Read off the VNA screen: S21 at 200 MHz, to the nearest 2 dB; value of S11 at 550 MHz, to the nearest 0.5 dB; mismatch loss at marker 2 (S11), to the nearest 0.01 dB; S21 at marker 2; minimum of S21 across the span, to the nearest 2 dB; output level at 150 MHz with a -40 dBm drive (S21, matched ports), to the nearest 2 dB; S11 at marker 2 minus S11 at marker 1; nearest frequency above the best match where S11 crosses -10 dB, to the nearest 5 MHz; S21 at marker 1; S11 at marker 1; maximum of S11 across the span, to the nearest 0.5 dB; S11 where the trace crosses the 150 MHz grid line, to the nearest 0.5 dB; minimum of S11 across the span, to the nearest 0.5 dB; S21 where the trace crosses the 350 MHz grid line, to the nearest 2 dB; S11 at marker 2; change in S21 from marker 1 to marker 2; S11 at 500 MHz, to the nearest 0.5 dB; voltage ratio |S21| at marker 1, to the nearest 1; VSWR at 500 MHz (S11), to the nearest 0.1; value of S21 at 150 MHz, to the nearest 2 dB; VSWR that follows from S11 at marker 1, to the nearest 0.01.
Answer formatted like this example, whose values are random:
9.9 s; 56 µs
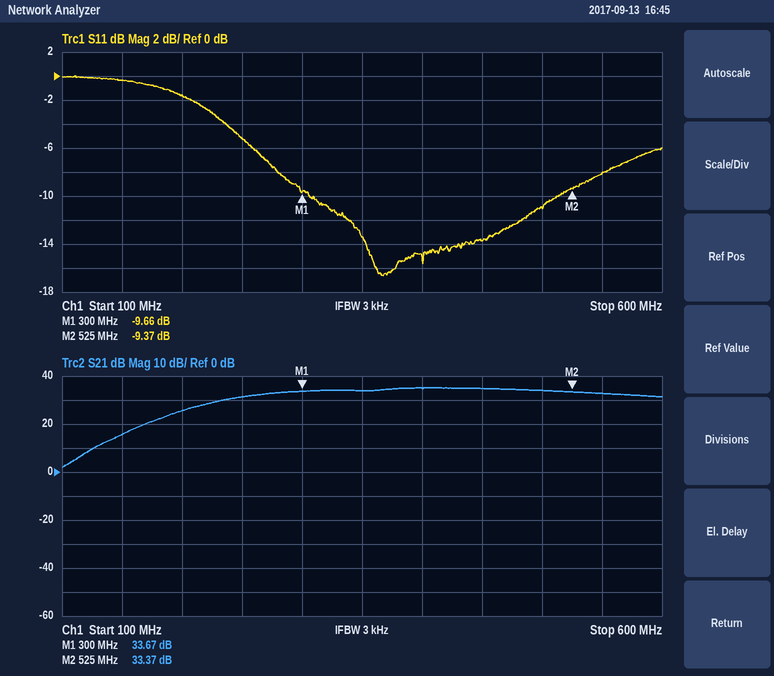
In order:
26 dB; -8.0 dB; 0.53 dB; 33.37 dB; 2 dB; -24 dBm; 0.29 dB; 515 MHz; 33.67 dB; -9.66 dB; 0.0 dB; -0.5 dB; -16.5 dB; 34 dB; -9.37 dB; -0.30 dB; -11.0 dB; 48; 1.8; 16 dB; 1.98
